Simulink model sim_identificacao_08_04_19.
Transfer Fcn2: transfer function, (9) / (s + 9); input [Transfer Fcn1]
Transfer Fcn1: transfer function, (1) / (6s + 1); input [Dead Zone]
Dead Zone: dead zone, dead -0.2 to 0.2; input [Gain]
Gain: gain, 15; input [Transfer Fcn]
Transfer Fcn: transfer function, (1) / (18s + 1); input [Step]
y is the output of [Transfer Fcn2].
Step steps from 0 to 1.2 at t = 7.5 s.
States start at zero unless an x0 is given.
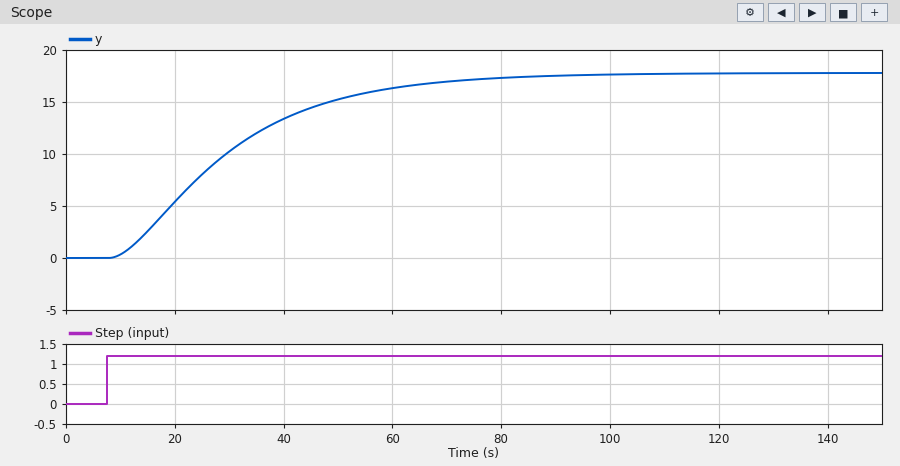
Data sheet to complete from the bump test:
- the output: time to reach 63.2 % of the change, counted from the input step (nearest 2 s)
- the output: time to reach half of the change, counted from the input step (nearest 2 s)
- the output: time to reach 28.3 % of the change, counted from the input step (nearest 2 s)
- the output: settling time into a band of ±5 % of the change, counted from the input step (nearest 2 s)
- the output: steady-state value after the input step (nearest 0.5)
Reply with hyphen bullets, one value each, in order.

- 26 s
- 20 s
- 12 s
- 62 s
- 18.0
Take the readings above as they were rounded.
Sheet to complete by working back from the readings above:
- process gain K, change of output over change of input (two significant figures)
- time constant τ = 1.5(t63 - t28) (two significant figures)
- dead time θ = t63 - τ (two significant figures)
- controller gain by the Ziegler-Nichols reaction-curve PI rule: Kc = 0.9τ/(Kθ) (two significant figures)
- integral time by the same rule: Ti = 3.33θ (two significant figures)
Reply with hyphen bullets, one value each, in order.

- 15
- 21 s
- 5.0 s
- 0.25
- 17 s
